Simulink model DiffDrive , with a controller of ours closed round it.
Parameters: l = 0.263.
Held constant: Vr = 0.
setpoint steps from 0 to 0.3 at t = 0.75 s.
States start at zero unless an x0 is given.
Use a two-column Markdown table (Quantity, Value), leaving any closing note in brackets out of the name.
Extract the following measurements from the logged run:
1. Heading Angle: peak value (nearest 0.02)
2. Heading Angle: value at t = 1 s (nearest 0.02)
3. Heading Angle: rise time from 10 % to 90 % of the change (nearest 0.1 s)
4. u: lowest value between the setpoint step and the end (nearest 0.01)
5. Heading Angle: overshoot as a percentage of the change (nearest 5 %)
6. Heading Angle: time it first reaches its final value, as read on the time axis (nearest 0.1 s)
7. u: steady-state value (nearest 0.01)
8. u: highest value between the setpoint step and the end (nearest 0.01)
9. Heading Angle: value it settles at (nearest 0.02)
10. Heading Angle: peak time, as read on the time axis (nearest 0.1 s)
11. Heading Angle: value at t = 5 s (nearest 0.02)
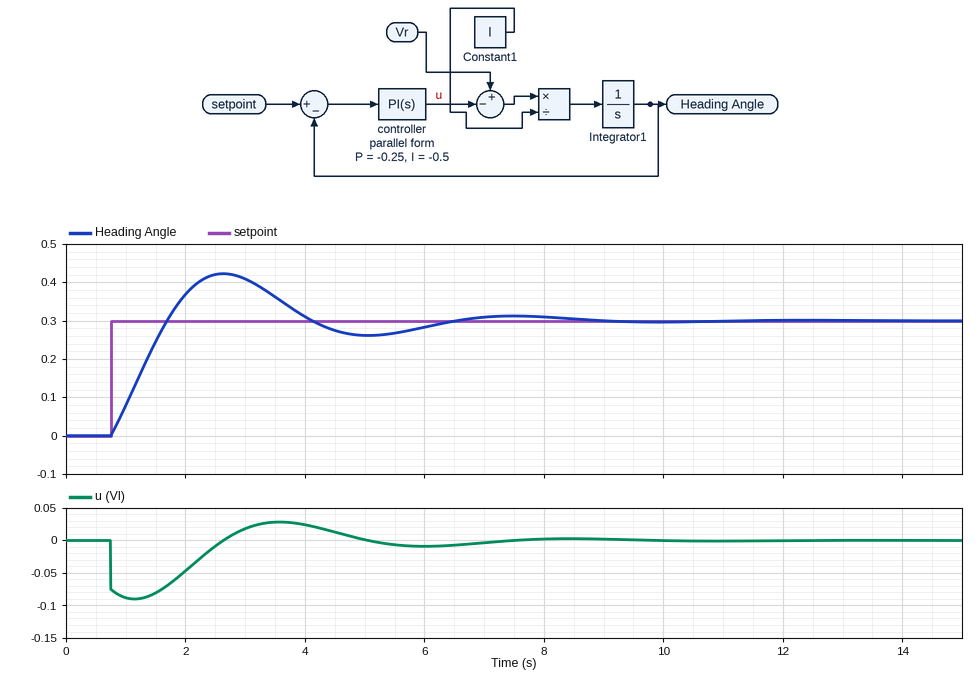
| Quantity | Value |
|---|---|
| Heading Angle: peak value | 0.42 |
| Heading Angle: value at t = 1 s | 0.08 |
| Heading Angle: rise time from 10 % to 90 % of the change | 0.7 s |
| u: lowest value between the setpoint step and the end | -0.09 |
| Heading Angle: overshoot as a percentage of the change | 40 % |
| Heading Angle: time it first reaches its final value, as read on the time axis | 1.7 s |
| u: steady-state value | 0.00 |
| u: highest value between the setpoint step and the end | 0.03 |
| Heading Angle: value it settles at | 0.30 |
| Heading Angle: peak time, as read on the time axis | 2.6 s |
| Heading Angle: value at t = 5 s | 0.26 |
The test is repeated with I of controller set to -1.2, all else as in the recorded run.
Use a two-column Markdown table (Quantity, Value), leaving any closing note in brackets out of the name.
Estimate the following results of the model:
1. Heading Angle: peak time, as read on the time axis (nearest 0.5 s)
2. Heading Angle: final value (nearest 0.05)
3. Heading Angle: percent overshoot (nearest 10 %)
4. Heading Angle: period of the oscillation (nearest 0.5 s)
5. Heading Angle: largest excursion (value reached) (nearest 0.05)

| Quantity | Value |
|---|---|
| Heading Angle: peak time, as read on the time axis | 2.0 s |
| Heading Angle: final value | 0.30 |
| Heading Angle: percent overshoot | 50 % |
| Heading Angle: period of the oscillation | 3.0 s |
| Heading Angle: largest excursion (value reached) | 0.45 |
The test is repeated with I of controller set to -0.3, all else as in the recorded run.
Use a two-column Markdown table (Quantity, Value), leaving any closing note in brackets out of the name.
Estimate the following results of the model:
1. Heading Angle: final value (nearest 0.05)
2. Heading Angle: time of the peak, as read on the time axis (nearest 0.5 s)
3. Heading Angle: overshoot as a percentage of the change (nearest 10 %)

| Quantity | Value |
|---|---|
| Heading Angle: final value | 0.30 |
| Heading Angle: time of the peak, as read on the time axis | 3.0 s |
| Heading Angle: overshoot as a percentage of the change | 30 % |
